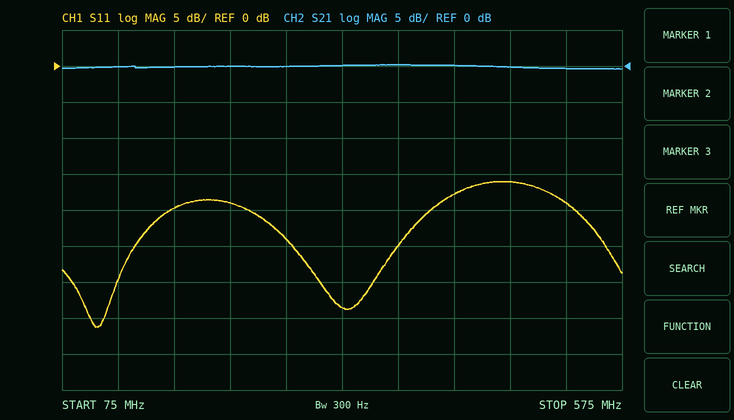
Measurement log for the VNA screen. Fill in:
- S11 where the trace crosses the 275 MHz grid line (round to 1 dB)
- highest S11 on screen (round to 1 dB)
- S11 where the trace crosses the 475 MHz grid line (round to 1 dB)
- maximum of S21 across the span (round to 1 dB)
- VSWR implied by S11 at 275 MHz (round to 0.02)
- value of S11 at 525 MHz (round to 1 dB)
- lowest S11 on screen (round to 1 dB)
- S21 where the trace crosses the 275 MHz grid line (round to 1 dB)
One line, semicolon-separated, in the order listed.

-24 dB; -16 dB; -16 dB; 0 dB; 1.14; -19 dB; -36 dB; 0 dB
